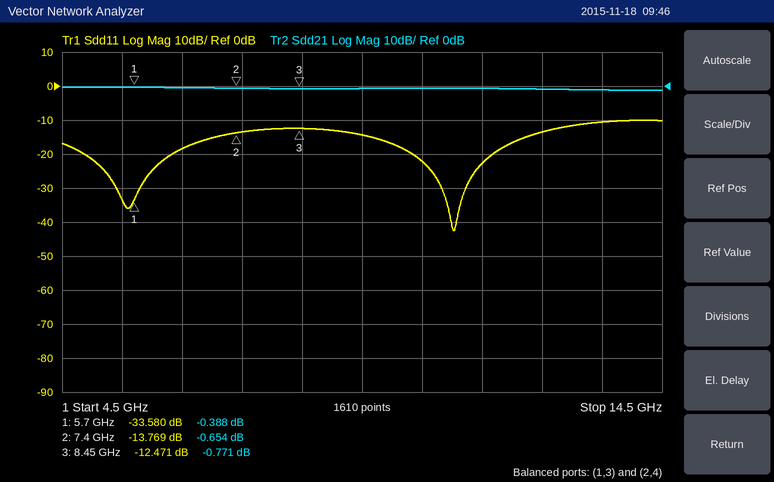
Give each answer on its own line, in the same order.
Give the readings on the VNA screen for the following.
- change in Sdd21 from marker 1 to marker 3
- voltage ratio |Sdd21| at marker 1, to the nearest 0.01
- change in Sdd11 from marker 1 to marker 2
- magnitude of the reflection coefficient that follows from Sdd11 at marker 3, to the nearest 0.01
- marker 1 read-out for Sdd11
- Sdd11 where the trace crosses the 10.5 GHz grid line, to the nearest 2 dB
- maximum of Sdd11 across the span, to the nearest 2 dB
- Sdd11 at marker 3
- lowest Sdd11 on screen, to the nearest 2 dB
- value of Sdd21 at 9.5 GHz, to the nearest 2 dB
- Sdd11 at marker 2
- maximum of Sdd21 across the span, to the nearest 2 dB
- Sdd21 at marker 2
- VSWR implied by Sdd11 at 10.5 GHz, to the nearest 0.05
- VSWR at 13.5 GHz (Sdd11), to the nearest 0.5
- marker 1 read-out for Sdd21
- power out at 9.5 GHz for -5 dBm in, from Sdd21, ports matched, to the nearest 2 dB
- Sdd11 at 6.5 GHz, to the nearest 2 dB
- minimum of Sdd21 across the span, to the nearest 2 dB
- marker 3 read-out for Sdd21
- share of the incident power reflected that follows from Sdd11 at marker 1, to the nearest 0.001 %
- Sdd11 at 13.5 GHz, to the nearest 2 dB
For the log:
-0.383 dB
0.96
19.811 dB
0.24
-33.580 dB
-22 dB
-10 dB
-12.471 dB
-42 dB
0 dB
-13.769 dB
0 dB
-0.654 dB
1.15
2.0
-0.388 dB
-6 dBm
-18 dB
-2 dB
-0.771 dB
0.044 %
-10 dB
